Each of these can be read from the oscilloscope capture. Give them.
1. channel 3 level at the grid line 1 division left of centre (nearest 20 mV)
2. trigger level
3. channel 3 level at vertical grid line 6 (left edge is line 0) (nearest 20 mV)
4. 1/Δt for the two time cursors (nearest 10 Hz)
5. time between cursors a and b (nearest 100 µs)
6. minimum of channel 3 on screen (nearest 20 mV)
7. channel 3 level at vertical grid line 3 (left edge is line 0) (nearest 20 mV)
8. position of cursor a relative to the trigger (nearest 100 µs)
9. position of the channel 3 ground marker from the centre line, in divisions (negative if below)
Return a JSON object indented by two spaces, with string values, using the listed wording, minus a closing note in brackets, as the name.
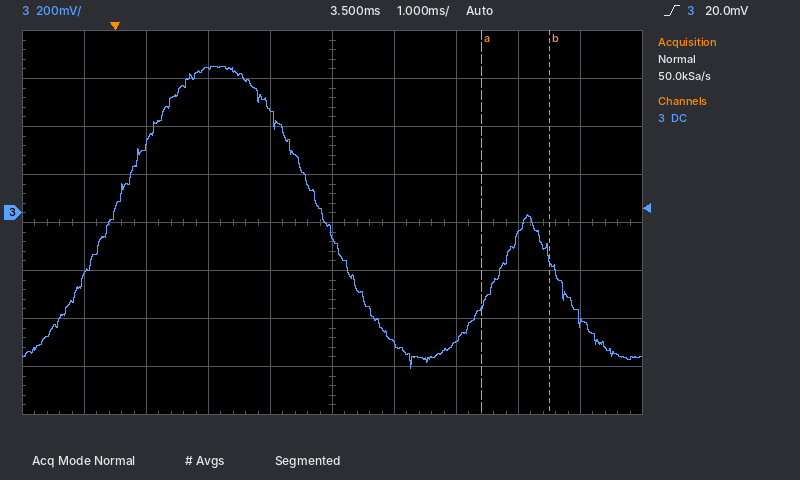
{
  "channel 3 level at the grid line 1 division left of centre": "440 mV",
  "trigger level": "20.0 mV",
  "channel 3 level at vertical grid line 6 (left edge is line 0)": "-540 mV",
  "1/Δt for the two time cursors": "910 Hz",
  "time between cursors a and b": "1.1 ms",
  "minimum of channel 3 on screen": "-640 mV",
  "channel 3 level at vertical grid line 3 (left edge is line 0)": "600 mV",
  "position of cursor a relative to the trigger": "+5.9 ms",
  "position of the channel 3 ground marker from the centre line, in divisions": "+0.2 div"
}
